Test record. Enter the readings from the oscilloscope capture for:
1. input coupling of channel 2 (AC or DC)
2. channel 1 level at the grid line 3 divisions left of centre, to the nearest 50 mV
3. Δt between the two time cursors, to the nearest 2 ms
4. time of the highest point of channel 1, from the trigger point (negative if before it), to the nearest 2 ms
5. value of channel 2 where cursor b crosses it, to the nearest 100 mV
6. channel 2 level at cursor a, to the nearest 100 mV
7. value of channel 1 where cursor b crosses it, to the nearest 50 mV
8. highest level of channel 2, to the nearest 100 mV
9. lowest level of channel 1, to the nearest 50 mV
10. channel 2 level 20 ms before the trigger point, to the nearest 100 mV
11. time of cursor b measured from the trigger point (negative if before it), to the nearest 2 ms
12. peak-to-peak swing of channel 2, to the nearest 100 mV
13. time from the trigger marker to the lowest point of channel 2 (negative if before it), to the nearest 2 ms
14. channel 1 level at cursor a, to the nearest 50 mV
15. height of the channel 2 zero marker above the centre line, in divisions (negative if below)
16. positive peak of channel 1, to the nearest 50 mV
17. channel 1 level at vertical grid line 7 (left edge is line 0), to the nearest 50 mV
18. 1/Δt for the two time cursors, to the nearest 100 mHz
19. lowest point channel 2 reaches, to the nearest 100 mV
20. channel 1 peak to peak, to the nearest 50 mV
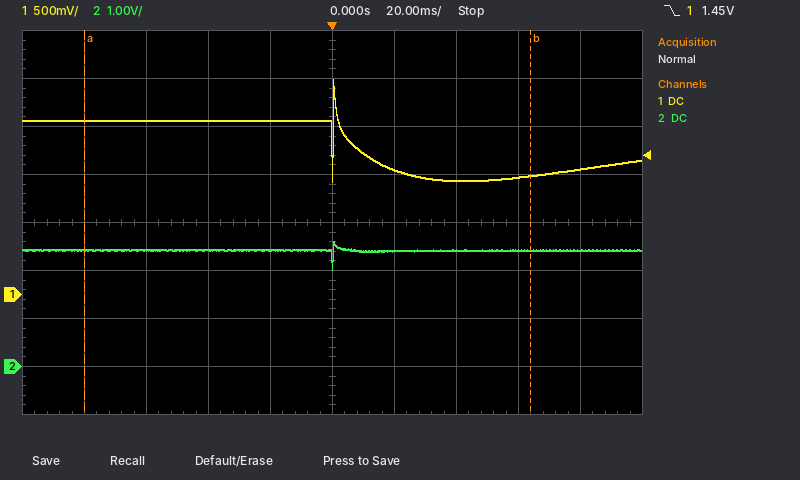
DC
1.80 V
144 ms
0 ms
2.4 V
2.4 V
1.25 V
2.6 V
1.20 V
2.4 V
+64 ms
600 mV
0 ms
1.80 V
-3.0 div
2.25 V
1.20 V
6.9 Hz
2.0 V
1.05 V
